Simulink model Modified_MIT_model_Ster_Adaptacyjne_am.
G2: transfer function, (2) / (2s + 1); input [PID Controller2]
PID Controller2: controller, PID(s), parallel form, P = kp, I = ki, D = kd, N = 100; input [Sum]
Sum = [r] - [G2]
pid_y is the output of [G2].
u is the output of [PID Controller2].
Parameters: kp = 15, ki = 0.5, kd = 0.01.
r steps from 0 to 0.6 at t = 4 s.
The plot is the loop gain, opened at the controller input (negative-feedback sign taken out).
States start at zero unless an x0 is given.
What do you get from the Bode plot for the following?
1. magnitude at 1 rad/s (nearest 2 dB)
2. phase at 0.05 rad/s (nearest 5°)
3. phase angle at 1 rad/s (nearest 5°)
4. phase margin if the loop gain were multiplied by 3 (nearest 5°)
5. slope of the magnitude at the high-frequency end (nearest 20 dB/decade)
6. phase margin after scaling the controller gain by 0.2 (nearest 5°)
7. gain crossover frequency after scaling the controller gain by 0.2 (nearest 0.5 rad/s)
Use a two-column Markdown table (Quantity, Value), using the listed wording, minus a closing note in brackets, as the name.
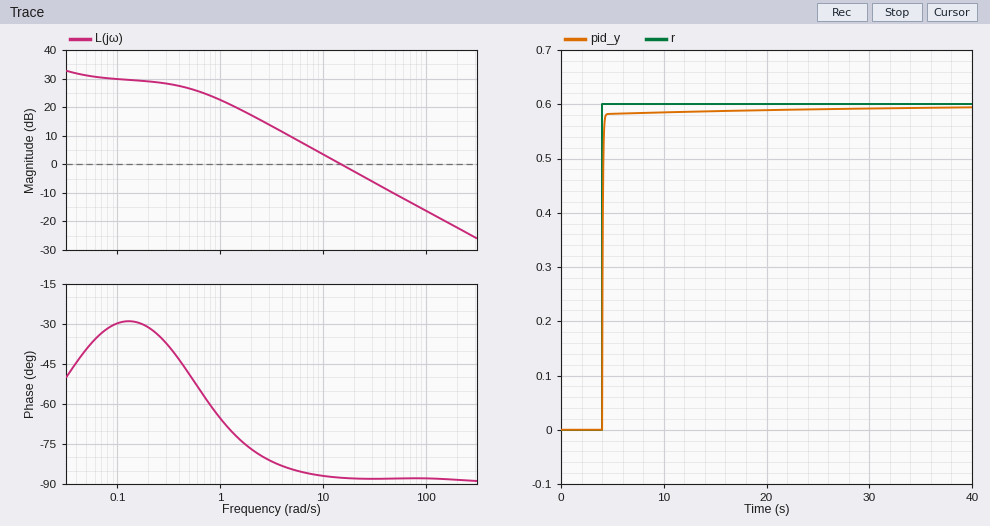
| Quantity | Value |
|---|---|
| magnitude at 1 rad/s | 22 dB |
| phase at 0.05 rad/s | -40° |
| phase angle at 1 rad/s | -65° |
| phase margin if the loop gain were multiplied by 3 | 90° |
| slope of the magnitude at the high-frequency end | -20 dB/decade |
| phase margin after scaling the controller gain by 0.2 | 100° |
| gain crossover frequency after scaling the controller gain by 0.2 | 3.0 rad/s |
